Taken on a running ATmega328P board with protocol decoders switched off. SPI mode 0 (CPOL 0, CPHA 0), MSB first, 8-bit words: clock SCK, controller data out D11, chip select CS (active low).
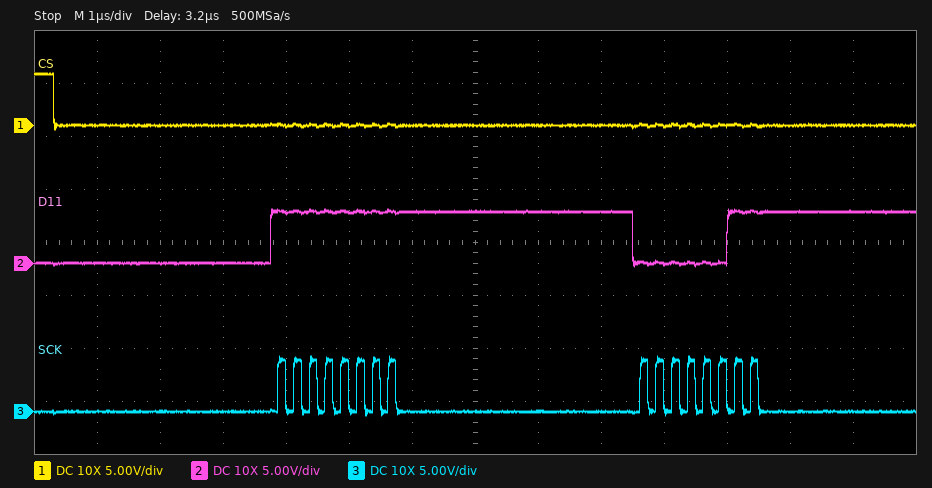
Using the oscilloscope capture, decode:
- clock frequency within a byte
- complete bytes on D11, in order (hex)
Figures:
4 MHz
0xFF 0x03
